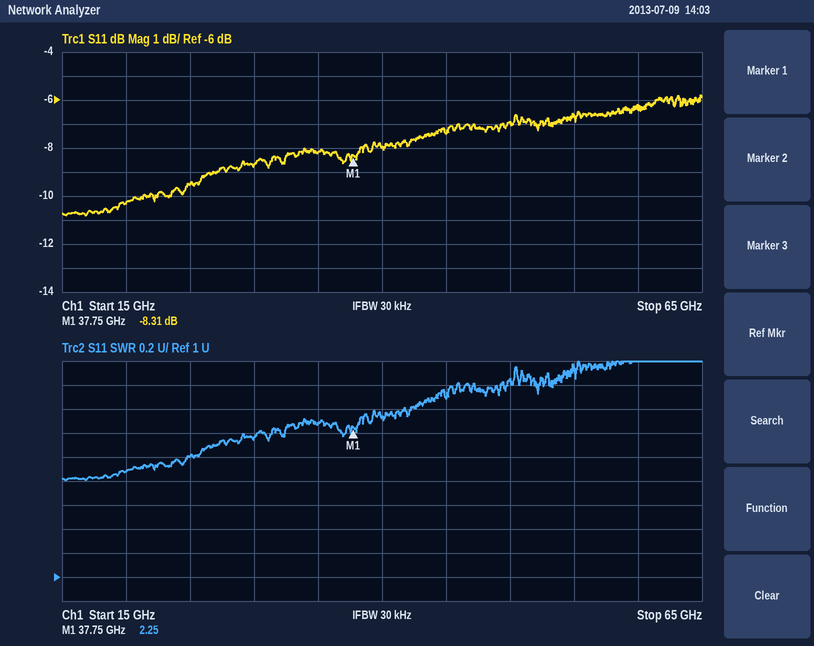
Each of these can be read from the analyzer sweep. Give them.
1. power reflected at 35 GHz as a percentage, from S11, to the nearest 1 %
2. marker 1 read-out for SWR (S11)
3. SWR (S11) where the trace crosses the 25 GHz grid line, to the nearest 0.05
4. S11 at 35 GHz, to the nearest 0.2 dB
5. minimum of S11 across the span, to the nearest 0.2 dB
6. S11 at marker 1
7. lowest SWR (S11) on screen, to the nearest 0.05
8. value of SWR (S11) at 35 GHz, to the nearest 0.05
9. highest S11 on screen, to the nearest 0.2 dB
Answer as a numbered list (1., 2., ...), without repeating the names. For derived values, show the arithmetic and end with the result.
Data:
1. 10^(-8.2/10) ≈ 15 %
2. 2.25
3. 2.00
4. -8.2 dB
5. -10.8 dB
6. -8.31 dB
7. 1.80
8. 2.30
9. -5.8 dB
